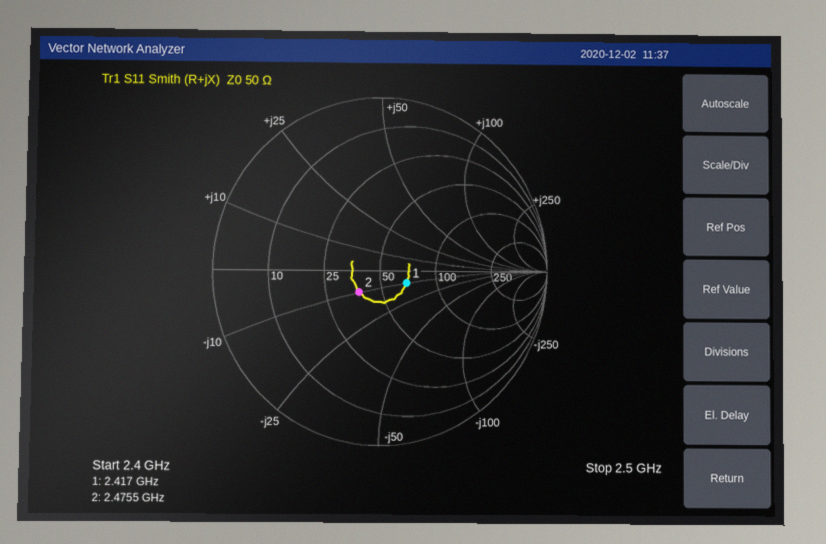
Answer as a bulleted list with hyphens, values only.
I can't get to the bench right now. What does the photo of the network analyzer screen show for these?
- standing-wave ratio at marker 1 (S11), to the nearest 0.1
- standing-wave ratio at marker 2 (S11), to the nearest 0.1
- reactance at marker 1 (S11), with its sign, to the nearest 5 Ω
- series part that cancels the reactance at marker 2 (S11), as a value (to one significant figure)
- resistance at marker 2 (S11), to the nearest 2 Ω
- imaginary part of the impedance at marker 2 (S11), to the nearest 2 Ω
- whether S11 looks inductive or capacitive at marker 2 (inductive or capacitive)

- 1.4
- 1.4
- -10 Ω
- 600 pH
- 38 Ω
- -10 Ω
- capacitive
